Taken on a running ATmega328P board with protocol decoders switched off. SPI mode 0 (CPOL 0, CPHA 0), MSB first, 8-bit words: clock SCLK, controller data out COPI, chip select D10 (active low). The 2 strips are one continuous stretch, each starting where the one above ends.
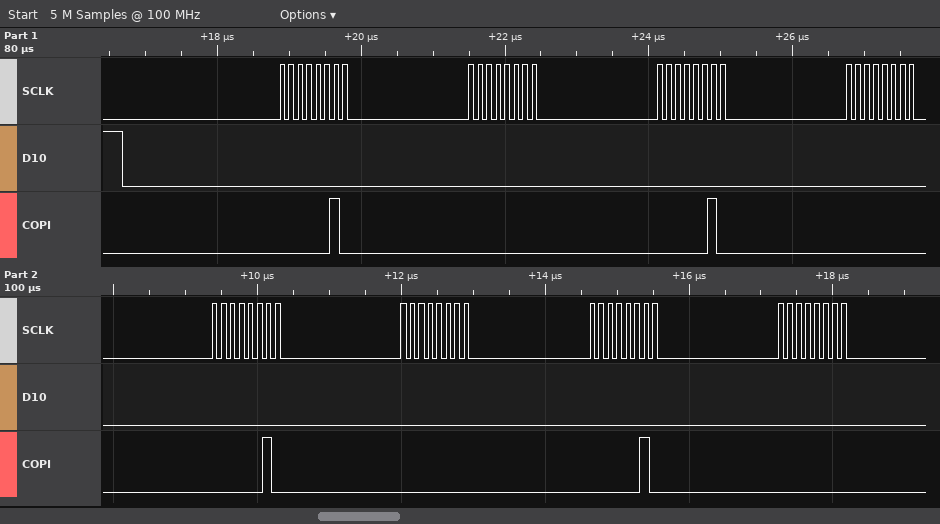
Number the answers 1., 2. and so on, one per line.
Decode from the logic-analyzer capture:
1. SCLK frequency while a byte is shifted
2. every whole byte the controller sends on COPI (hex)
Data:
1. 8 MHz
2. 0x02 0x00 0x02 0x00 0x02 0x00 0x02 0x00
